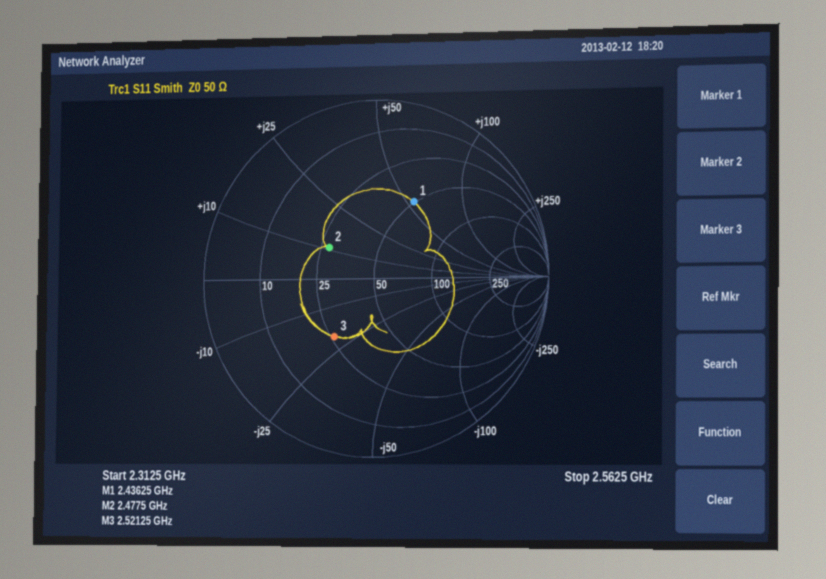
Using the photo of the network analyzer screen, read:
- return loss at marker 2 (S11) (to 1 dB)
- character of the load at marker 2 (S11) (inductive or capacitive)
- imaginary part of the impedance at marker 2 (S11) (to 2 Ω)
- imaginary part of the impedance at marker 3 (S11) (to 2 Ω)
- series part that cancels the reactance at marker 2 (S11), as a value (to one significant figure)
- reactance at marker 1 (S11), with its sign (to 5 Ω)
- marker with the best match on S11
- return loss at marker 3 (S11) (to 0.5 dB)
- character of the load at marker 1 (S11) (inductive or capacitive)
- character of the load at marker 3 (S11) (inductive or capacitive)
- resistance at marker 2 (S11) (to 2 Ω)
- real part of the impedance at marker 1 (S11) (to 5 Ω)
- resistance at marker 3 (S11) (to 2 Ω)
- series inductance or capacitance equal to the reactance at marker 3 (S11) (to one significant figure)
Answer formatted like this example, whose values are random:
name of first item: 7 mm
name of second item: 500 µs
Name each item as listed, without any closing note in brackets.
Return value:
return loss at marker 2 (S11): 10 dB
character of the load at marker 2 (S11): inductive
imaginary part of the impedance at marker 2 (S11): +10 Ω
imaginary part of the impedance at marker 3 (S11): -20 Ω
series part that cancels the reactance at marker 2 (S11), as a value: 6 pF
reactance at marker 1 (S11), with its sign: +55 Ω
marker with the best match on S11: marker 2
return loss at marker 3 (S11): 8.0 dB
character of the load at marker 1 (S11): inductive
character of the load at marker 3 (S11): capacitive
resistance at marker 2 (S11): 28 Ω
real part of the impedance at marker 1 (S11): 50 Ω
resistance at marker 3 (S11): 26 Ω
series inductance or capacitance equal to the reactance at marker 3 (S11): 3 pF
